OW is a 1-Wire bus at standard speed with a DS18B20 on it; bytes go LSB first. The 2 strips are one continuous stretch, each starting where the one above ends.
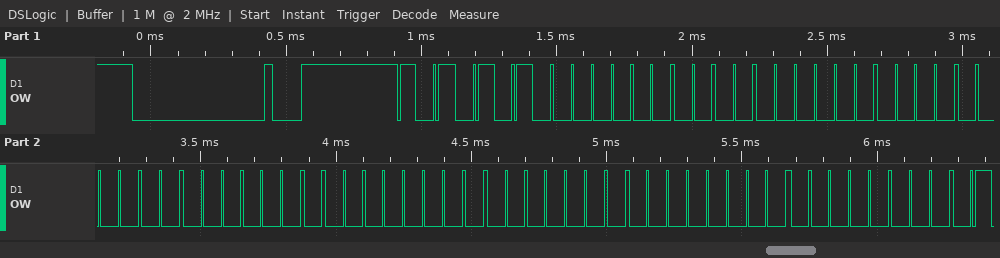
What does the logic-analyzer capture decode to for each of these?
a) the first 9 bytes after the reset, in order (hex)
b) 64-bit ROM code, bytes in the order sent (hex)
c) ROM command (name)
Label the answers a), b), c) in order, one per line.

a) 55 00 00 00 00 00 00 00 00
b) 00 00 00 00 00 00 00 00
c) Match ROM
